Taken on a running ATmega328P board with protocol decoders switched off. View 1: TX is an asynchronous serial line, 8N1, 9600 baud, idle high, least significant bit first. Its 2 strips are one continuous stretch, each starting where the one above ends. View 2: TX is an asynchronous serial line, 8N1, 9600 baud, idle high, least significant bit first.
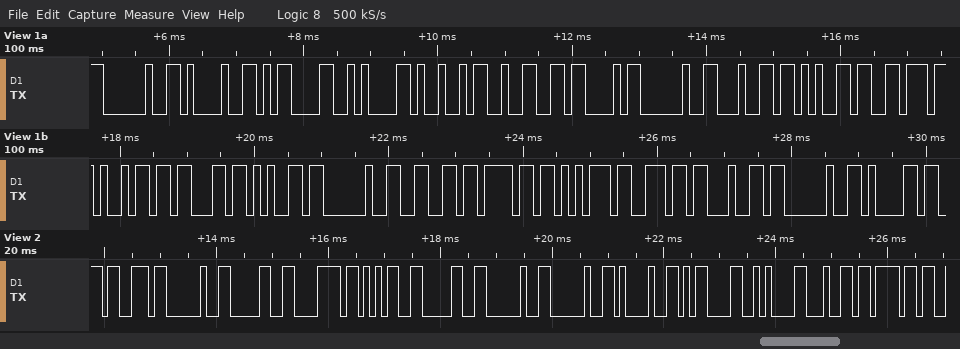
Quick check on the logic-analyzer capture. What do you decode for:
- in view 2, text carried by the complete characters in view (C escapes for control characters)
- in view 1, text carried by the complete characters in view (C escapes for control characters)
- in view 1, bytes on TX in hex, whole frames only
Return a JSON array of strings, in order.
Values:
["\"s 0x50  !\\r\\ndo\"", "\" !\\r\\nI2C device found a\"", "0x20 0x21 0x0D 0x0A 0x49 0x32 0x43 0x20 0x64 0x65 0x76 0x69 0x63 0x65 0x20 0x66 0x6F 0x75 0x6E 0x64 0x20 0x61"]
